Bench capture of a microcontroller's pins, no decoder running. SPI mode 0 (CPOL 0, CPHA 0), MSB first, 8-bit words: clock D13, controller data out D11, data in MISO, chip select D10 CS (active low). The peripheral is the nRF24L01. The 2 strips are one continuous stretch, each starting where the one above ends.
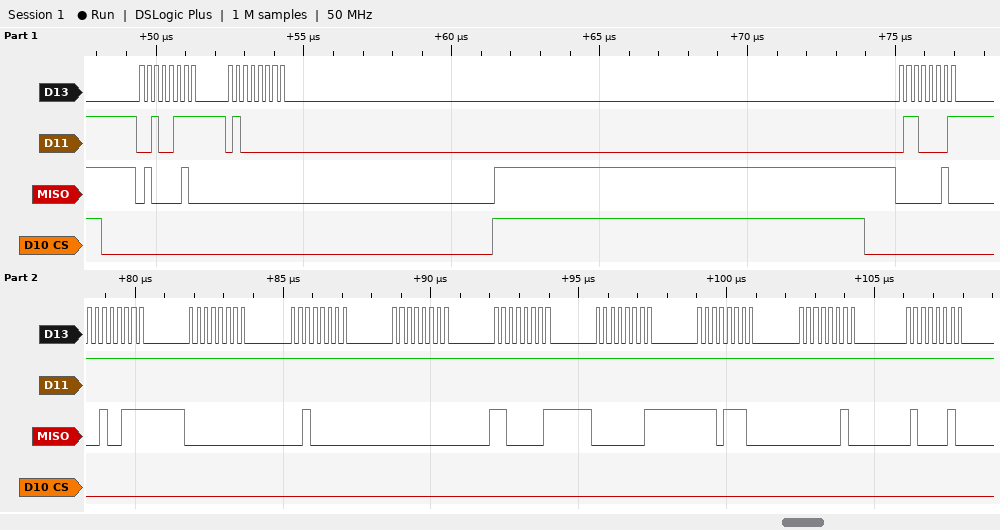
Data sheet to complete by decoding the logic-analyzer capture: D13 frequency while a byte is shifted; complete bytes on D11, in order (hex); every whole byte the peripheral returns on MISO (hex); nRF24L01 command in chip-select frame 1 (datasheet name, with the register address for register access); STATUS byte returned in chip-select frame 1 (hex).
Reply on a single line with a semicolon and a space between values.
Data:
4 MHz; 27 40 61 FF FF FF FF FF FF FF FF FF; 42 00 02 27 00 20 00 C1 01 EE 02 42; W_REGISTER 0x07; 0x42
